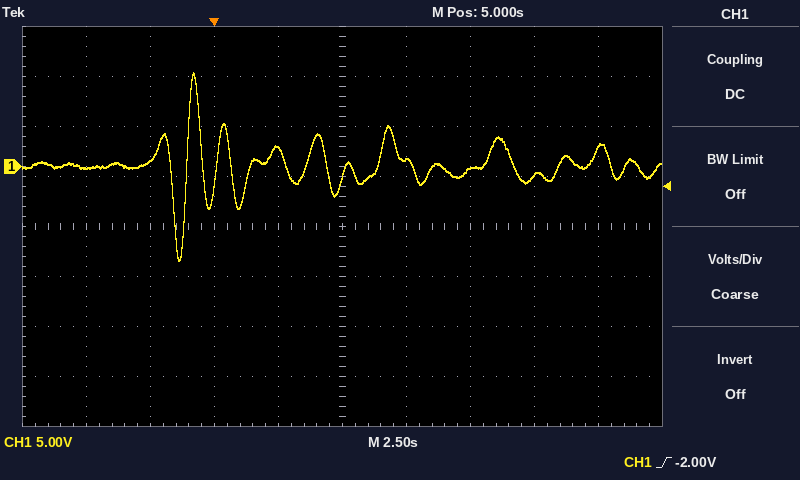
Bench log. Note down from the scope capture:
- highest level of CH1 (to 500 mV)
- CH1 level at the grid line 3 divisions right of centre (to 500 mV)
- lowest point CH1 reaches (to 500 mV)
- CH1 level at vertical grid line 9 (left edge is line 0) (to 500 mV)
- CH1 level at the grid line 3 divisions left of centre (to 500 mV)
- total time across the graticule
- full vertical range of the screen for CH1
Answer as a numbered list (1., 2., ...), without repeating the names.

1. 9.5 V
2. -1.0 V
3. -9.5 V
4. 2.0 V
5. 500 mV
6. 25 s
7. 40 V
